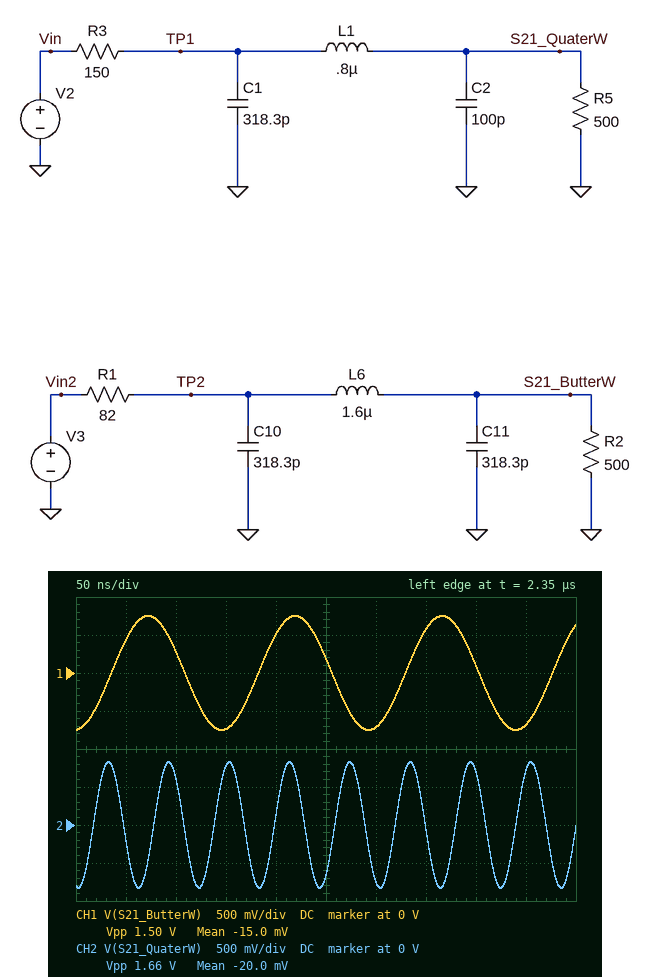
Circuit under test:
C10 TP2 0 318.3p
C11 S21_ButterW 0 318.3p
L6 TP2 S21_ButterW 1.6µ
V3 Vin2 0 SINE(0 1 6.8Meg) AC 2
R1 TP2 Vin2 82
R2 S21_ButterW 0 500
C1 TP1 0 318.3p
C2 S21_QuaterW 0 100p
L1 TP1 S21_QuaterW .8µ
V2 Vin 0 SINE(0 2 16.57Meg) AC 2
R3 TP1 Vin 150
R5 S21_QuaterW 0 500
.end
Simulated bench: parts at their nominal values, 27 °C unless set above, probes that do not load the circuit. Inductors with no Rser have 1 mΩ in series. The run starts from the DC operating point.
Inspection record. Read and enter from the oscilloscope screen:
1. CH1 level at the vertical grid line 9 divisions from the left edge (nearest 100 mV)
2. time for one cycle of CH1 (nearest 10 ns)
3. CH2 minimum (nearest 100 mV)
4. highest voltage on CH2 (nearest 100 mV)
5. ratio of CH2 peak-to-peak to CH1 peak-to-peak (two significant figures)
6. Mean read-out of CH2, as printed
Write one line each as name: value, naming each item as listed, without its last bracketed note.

CH1 level at the vertical grid line 9 divisions from the left edge: -700 mV
time for one cycle of CH1: 150 ns
CH2 minimum: -800 mV
highest voltage on CH2: 800 mV
ratio of CH2 peak-to-peak to CH1 peak-to-peak: 1.1
Mean read-out of CH2, as printed: -20.0 mV
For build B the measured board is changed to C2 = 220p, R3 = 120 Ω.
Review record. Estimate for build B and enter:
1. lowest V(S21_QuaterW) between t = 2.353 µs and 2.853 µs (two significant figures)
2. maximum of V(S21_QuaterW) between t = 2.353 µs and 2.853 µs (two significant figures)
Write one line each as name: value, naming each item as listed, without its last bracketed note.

lowest V(S21_QuaterW) between t = 2.353 µs and 2.853 µs: -1.3 V
maximum of V(S21_QuaterW) between t = 2.353 µs and 2.853 µs: 1.3 V
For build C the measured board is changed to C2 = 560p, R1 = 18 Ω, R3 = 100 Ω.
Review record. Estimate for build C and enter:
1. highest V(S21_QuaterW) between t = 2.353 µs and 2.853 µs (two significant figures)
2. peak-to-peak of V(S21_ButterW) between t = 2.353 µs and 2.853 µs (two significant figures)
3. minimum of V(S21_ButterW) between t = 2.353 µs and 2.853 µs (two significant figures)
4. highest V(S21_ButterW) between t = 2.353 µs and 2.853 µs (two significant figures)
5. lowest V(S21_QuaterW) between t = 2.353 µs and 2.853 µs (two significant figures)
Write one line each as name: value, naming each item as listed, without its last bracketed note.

highest V(S21_QuaterW) between t = 2.353 µs and 2.853 µs: 250 mV
peak-to-peak of V(S21_ButterW) between t = 2.353 µs and 2.853 µs: 4.9 V
minimum of V(S21_ButterW) between t = 2.353 µs and 2.853 µs: -2.5 V
highest V(S21_ButterW) between t = 2.353 µs and 2.853 µs: 2.5 V
lowest V(S21_QuaterW) between t = 2.353 µs and 2.853 µs: -250 mV
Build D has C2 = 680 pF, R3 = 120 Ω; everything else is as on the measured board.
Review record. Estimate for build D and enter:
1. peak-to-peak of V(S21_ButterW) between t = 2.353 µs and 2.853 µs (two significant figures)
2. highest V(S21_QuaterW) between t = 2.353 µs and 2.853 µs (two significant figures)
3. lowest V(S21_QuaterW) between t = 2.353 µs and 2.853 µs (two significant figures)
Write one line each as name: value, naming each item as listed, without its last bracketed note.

peak-to-peak of V(S21_ButterW) between t = 2.353 µs and 2.853 µs: 1.5 V
highest V(S21_QuaterW) between t = 2.353 µs and 2.853 µs: 170 mV
lowest V(S21_QuaterW) between t = 2.353 µs and 2.853 µs: -170 mV
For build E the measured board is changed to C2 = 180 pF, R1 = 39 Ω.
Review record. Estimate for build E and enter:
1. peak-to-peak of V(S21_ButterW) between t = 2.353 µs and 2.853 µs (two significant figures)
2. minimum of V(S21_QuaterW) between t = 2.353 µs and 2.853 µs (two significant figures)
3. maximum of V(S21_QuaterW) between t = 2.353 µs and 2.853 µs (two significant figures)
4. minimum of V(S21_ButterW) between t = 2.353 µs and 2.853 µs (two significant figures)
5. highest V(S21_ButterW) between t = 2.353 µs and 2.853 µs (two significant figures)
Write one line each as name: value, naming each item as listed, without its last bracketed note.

peak-to-peak of V(S21_ButterW) between t = 2.353 µs and 2.853 µs: 2.8 V
minimum of V(S21_QuaterW) between t = 2.353 µs and 2.853 µs: -1.8 V
maximum of V(S21_QuaterW) between t = 2.353 µs and 2.853 µs: 1.8 V
minimum of V(S21_ButterW) between t = 2.353 µs and 2.853 µs: -1.4 V
highest V(S21_ButterW) between t = 2.353 µs and 2.853 µs: 1.4 V
